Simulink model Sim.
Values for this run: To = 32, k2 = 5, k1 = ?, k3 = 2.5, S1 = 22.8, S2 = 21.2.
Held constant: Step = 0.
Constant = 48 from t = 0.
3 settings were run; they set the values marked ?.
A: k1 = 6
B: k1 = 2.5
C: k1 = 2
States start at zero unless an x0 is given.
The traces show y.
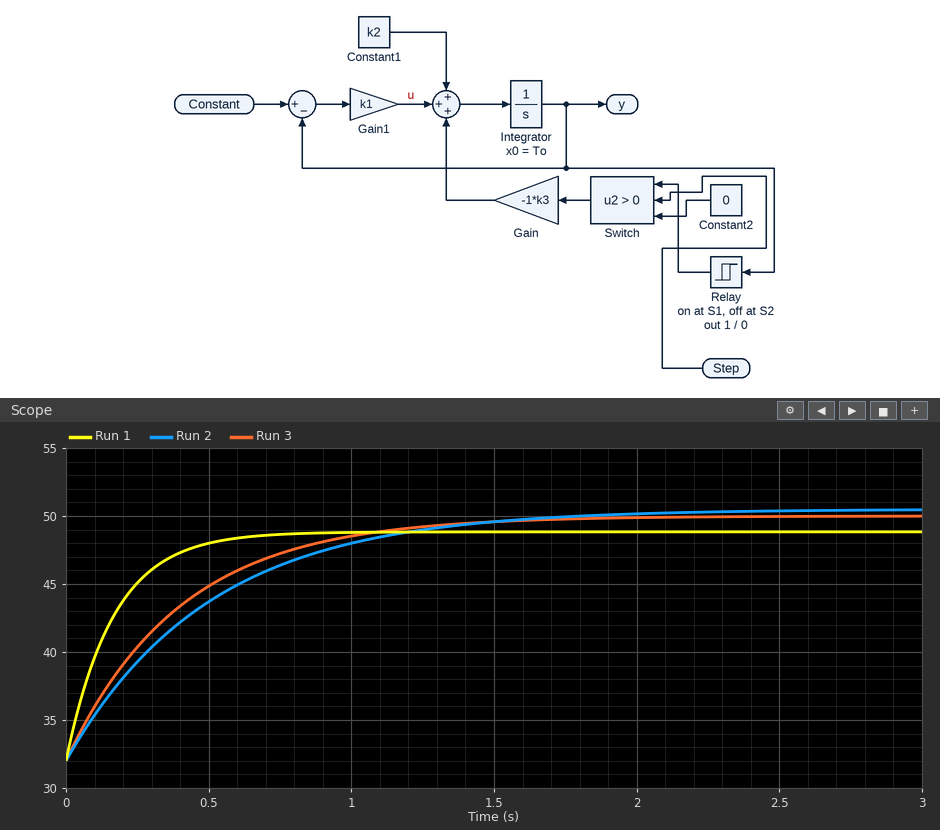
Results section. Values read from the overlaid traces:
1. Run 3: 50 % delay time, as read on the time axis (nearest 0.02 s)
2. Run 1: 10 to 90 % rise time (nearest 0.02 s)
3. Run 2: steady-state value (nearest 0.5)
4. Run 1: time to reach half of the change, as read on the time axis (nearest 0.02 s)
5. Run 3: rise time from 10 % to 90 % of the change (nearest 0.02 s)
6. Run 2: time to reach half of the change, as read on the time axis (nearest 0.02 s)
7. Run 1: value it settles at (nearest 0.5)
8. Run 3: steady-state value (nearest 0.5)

0.28 s
0.36 s
50.5
0.12 s
0.88 s
0.34 s
49.0
50.0
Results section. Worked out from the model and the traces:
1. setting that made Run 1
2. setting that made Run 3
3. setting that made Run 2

A
B
C
